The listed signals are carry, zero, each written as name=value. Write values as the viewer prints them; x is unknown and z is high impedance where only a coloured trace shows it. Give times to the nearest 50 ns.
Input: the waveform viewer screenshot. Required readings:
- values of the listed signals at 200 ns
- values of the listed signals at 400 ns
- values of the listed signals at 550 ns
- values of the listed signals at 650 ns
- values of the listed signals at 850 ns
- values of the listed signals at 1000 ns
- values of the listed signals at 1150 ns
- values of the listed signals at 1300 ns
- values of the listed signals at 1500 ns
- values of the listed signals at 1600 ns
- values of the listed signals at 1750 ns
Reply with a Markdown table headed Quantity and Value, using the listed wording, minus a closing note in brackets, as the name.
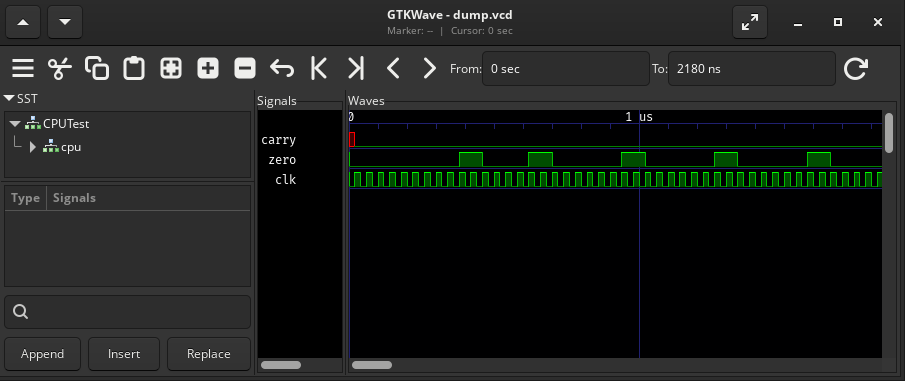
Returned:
| Quantity | Value |
|---|---|
| values of the listed signals at 200 ns | carry=0, zero=0 |
| values of the listed signals at 400 ns | carry=0, zero=1 |
| values of the listed signals at 550 ns | carry=0, zero=0 |
| values of the listed signals at 650 ns | carry=0, zero=1 |
| values of the listed signals at 850 ns | carry=0, zero=0 |
| values of the listed signals at 1000 ns | carry=0, zero=1 |
| values of the listed signals at 1150 ns | carry=0, zero=0 |
| values of the listed signals at 1300 ns | carry=0, zero=1 |
| values of the listed signals at 1500 ns | carry=0, zero=0 |
| values of the listed signals at 1600 ns | carry=0, zero=1 |
| values of the listed signals at 1750 ns | carry=0, zero=0 |
